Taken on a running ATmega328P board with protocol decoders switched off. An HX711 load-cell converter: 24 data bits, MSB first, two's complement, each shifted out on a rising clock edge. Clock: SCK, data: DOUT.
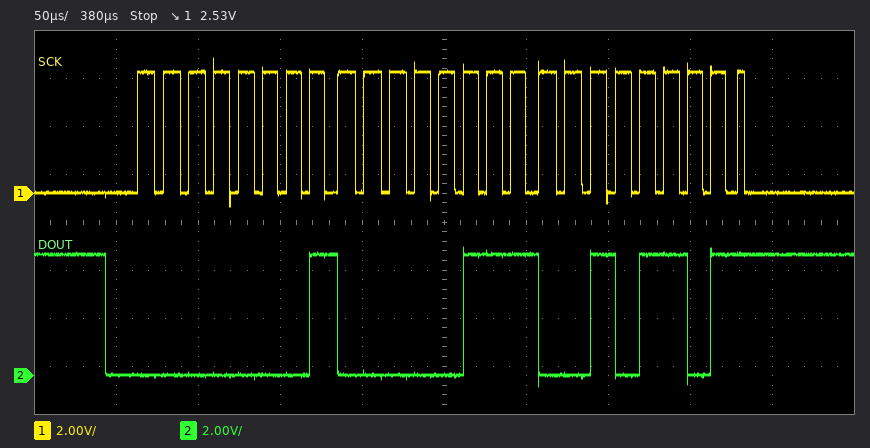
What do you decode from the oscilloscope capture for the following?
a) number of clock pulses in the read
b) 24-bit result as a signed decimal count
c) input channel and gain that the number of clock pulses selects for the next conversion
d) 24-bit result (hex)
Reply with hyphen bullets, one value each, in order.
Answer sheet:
- 25
- 67373
- channel A, gain 128
- 0x01072D
